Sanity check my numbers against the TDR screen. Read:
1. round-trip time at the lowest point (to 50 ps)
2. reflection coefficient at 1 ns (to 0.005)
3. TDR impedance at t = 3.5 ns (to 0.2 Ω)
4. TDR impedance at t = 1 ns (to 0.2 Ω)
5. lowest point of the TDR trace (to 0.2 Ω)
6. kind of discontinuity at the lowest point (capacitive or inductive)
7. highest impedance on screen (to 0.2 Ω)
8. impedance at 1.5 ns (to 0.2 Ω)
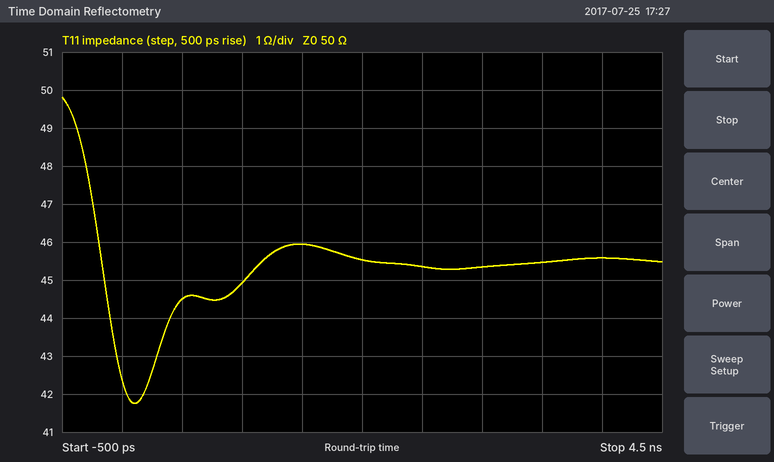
100 ps
-0.055
45.4 Ω
45.0 Ω
41.8 Ω
capacitive
49.8 Ω
46.0 Ω
